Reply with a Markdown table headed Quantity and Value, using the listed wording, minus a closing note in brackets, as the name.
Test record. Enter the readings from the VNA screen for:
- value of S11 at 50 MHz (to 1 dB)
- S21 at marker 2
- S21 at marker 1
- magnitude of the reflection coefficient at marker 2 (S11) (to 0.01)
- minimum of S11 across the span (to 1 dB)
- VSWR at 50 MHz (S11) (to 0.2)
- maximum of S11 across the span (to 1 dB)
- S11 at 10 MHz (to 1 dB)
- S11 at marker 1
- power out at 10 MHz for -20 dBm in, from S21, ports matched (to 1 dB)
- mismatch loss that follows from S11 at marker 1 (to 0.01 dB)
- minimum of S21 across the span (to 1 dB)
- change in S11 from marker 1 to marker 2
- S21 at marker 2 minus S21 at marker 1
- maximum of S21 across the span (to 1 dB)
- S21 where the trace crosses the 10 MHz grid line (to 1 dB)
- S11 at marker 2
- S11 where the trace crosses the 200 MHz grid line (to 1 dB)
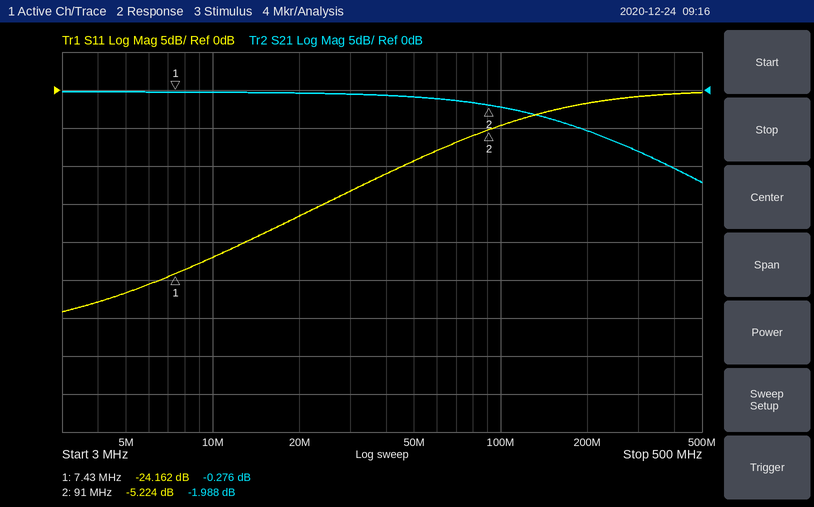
| Quantity | Value |
|---|---|
| value of S11 at 50 MHz | -9 dB |
| S21 at marker 2 | -1.988 dB |
| S21 at marker 1 | -0.276 dB |
| magnitude of the reflection coefficient at marker 2 (S11) | 0.55 |
| minimum of S11 across the span | -29 dB |
| VSWR at 50 MHz (S11) | 2.0 |
| maximum of S11 across the span | 0 dB |
| S11 at 10 MHz | -22 dB |
| S11 at marker 1 | -24.162 dB |
| power out at 10 MHz for -20 dBm in, from S21, ports matched | -20 dBm |
| mismatch loss that follows from S11 at marker 1 | 0.02 dB |
| minimum of S21 across the span | -12 dB |
| change in S11 from marker 1 to marker 2 | 18.938 dB |
| S21 at marker 2 minus S21 at marker 1 | -1.712 dB |
| maximum of S21 across the span | 0 dB |
| S21 where the trace crosses the 10 MHz grid line | 0 dB |
| S11 at marker 2 | -5.224 dB |
| S11 where the trace crosses the 200 MHz grid line | -2 dB |
